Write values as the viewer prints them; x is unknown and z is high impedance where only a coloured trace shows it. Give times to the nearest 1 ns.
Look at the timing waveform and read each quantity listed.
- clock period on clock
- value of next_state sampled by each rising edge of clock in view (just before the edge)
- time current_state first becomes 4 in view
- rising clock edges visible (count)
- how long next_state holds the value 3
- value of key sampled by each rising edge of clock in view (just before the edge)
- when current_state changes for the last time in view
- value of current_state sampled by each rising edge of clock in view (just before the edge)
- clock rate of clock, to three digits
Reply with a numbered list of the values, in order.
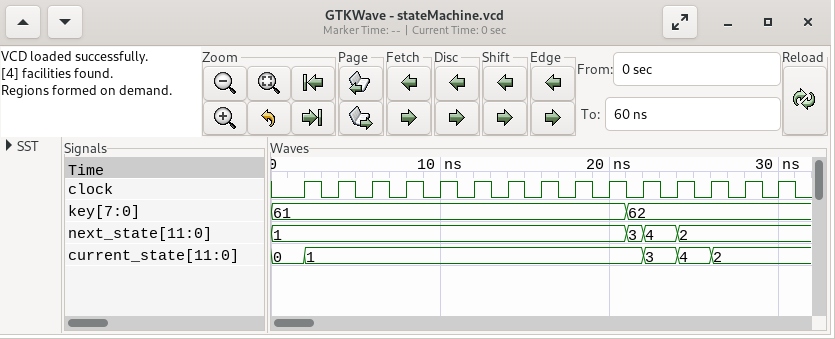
1. 2 ns
2. 1, 1, 1, 1, 1, 1, 1, 1, 1, 1, 3, 4, 2, 2, 2
3. 24 ns
4. 15
5. 1 ns
6. 61, 61, 61, 61, 61, 61, 61, 61, 61, 61, 62, 62, 62, 62, 62
7. 26 ns
8. 0, 1, 1, 1, 1, 1, 1, 1, 1, 1, 1, 3, 4, 2, 2
9. 500 MHz
